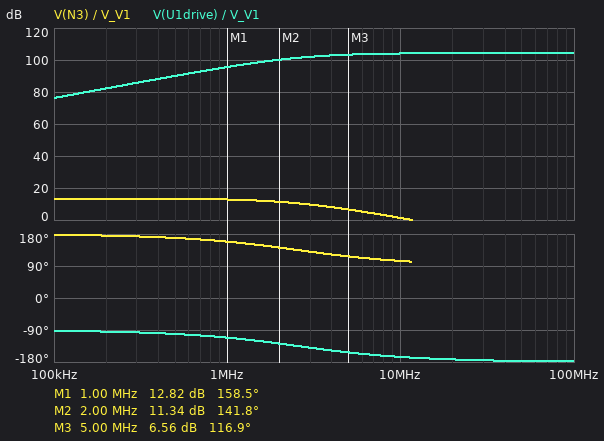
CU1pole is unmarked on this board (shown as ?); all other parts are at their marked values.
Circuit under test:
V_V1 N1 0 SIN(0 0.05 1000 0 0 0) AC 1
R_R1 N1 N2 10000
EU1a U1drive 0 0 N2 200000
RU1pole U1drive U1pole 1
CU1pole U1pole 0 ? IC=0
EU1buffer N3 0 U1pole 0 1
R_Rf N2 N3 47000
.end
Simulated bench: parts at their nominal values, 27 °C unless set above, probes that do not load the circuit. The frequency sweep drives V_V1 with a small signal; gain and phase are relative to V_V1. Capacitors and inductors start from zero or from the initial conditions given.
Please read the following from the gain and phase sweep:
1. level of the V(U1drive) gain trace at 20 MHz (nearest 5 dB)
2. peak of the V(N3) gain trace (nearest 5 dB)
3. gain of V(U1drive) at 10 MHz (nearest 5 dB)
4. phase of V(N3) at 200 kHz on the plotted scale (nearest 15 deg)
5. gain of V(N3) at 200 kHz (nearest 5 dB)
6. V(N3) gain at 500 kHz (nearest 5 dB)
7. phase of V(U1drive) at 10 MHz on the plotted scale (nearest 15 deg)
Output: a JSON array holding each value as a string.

["105 dB", "15 dB", "105 dB", "180 deg", "15 dB", "15 dB", "-165 deg"]
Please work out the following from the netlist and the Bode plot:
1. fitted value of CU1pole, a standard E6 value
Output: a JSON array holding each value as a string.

["2.2 mF"]
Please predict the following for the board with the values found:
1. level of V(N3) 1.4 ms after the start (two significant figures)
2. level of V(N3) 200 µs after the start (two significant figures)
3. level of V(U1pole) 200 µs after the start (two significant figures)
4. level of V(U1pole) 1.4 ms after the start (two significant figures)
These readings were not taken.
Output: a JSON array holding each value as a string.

["-140 mV", "-220 mV", "-220 mV", "-140 mV"]
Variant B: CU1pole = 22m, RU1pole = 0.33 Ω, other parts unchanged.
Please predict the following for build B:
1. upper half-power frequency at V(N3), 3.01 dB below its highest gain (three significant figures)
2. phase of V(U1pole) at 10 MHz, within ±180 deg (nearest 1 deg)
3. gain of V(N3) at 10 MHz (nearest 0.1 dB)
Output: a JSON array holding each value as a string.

["769 kHz", "94 deg", "-8.9 dB"]
